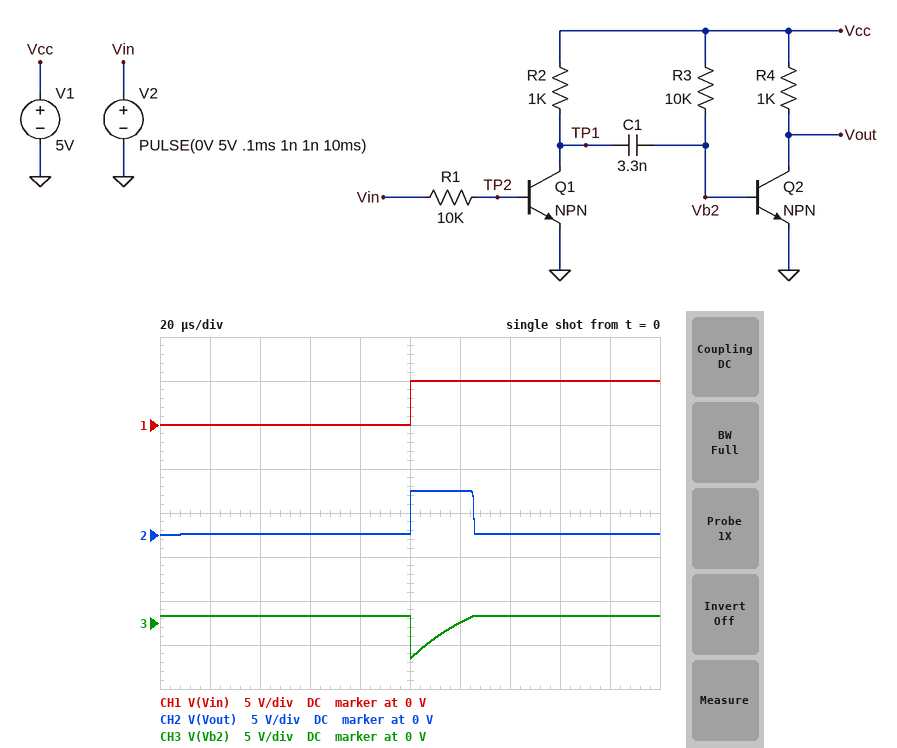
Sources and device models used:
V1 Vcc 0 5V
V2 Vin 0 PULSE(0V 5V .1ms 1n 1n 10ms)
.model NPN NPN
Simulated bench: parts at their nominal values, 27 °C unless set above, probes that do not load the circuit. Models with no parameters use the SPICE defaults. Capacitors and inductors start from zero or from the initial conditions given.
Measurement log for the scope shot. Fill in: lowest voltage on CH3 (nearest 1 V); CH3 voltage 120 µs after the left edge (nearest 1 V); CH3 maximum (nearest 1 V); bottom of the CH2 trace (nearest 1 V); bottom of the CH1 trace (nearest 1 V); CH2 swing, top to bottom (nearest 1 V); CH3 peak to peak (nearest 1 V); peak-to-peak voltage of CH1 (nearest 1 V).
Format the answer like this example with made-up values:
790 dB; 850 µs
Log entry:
-4 V; 0 V; 1 V; 0 V; 0 V; 5 V; 5 V; 5 V
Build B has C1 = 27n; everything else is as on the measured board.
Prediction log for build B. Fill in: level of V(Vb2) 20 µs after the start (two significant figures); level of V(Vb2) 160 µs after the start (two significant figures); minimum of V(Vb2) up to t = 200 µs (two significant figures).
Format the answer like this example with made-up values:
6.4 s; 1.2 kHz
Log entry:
830 mV; -2.2 V; -4.0 V
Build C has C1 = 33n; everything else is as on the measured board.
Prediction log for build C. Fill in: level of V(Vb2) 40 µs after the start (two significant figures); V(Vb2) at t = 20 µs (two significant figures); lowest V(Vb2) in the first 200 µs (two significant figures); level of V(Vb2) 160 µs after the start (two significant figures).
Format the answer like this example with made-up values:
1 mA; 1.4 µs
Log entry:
830 mV; 830 mV; -3.9 V; -2.4 V
